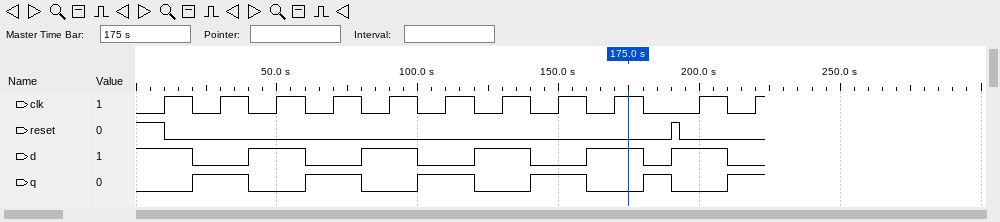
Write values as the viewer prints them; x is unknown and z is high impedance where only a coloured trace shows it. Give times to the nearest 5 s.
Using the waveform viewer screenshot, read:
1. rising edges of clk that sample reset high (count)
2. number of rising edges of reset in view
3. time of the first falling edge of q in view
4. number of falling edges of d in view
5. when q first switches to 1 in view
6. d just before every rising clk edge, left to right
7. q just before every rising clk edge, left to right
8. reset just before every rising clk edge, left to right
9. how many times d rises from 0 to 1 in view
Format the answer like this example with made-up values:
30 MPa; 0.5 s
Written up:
1; 1; 40 s; 6; 20 s; 1 0 1 0 1 0 1 0 1 1 0; 0 1 0 1 0 1 0 1 0 0 1; 1 0 0 0 0 0 0 0 0 0 0; 5
